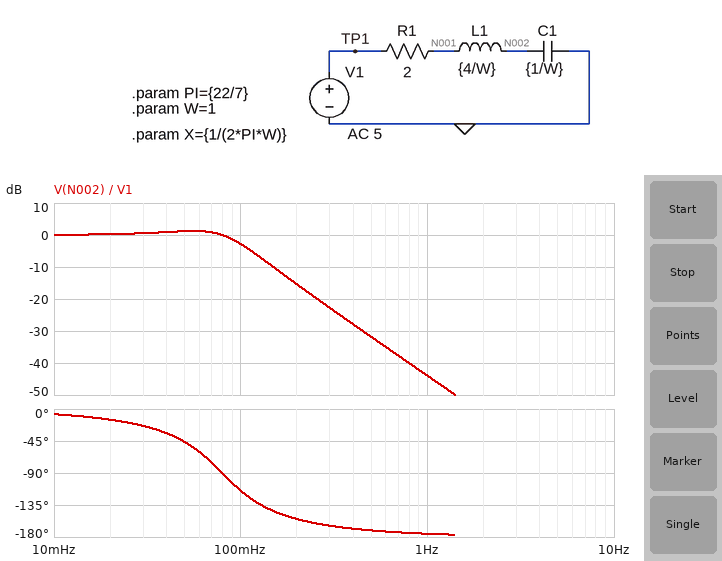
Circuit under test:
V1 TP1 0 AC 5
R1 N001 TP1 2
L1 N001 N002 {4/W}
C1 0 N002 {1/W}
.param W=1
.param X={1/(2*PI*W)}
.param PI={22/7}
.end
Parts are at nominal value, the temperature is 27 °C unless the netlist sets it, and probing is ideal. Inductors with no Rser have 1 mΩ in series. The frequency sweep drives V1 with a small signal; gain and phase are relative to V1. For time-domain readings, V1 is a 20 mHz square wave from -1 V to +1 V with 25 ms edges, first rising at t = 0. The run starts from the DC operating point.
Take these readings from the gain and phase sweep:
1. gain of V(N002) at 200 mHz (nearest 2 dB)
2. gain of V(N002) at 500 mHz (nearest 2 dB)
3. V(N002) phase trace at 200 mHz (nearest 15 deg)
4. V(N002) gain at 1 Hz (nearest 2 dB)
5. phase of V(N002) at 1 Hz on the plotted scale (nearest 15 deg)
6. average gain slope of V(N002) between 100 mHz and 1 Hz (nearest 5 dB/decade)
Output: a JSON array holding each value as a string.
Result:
["-16 dB", "-32 dB", "-150 deg", "-44 dB", "-180 deg", "-40 dB/decade"]
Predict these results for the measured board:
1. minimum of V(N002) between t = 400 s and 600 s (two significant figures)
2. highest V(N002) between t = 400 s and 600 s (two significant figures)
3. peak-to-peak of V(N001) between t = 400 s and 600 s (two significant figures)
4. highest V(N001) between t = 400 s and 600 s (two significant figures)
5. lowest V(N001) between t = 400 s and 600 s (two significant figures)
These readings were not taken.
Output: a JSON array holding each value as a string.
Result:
["-1.3 V", "1.3 V", "2.4 V", "1.2 V", "-1.2 V"]
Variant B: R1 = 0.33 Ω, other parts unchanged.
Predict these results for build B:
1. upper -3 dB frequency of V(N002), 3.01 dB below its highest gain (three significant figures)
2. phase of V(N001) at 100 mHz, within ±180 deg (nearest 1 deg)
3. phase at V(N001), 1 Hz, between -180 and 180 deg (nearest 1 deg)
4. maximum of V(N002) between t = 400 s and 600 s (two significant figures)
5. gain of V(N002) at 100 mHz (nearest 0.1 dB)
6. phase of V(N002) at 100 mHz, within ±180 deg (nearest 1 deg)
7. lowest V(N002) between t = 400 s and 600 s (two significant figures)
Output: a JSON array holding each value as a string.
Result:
["85.4 mHz", "20 deg", "1 deg", "2.1 V", "4.2 dB", "-160 deg", "-2.1 V"]
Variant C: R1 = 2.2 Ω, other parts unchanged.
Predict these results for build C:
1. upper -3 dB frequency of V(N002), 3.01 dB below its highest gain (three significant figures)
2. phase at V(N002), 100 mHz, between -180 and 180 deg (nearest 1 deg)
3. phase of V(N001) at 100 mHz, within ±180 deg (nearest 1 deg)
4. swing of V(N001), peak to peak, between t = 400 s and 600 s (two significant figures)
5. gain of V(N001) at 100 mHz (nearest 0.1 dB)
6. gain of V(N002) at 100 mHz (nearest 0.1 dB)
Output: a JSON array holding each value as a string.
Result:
["91.2 mHz", "-113 deg", "67 deg", "2.3 V", "-8.3 dB", "-3.5 dB"]
